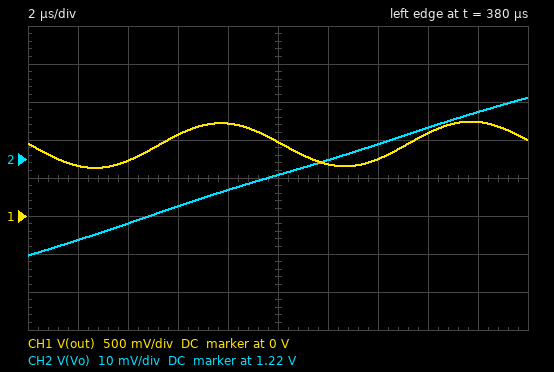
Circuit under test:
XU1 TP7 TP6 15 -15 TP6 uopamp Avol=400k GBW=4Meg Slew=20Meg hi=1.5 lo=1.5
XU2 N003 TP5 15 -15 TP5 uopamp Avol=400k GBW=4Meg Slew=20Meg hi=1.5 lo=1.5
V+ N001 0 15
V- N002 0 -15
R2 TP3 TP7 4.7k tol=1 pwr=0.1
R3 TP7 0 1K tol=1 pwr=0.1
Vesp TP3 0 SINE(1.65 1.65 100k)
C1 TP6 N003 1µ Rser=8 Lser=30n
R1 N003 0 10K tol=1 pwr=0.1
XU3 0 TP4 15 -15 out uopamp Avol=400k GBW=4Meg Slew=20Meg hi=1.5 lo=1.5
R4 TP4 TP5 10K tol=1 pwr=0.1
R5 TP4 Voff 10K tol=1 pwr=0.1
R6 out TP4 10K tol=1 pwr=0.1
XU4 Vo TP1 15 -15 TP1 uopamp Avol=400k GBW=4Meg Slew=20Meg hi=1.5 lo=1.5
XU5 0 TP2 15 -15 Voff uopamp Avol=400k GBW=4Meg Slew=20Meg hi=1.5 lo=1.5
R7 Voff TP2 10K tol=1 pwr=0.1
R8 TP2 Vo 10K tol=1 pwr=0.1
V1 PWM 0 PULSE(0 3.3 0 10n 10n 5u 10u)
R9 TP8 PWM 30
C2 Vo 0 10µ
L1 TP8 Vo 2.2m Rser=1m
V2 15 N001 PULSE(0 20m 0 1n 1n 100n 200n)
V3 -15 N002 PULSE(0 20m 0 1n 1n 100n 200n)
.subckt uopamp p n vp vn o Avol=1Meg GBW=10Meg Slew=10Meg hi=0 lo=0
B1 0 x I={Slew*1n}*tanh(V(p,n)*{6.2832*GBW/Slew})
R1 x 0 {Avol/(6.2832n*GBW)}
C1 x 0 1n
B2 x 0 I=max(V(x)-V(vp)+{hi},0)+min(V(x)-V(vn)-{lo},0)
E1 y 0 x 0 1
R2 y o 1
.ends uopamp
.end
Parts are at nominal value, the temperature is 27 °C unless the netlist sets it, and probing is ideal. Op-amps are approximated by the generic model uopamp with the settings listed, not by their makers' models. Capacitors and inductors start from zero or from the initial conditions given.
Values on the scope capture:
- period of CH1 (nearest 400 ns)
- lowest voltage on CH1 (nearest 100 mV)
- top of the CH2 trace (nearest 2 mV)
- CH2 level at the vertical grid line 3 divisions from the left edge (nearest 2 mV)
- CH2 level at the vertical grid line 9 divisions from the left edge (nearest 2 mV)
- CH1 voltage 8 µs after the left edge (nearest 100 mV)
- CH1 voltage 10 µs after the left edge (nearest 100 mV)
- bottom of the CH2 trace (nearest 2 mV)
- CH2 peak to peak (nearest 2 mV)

10.0 µs
600 mV
1.236 V
1.208 V
1.232 V
1.2 V
1.0 V
1.194 V
42 mV
